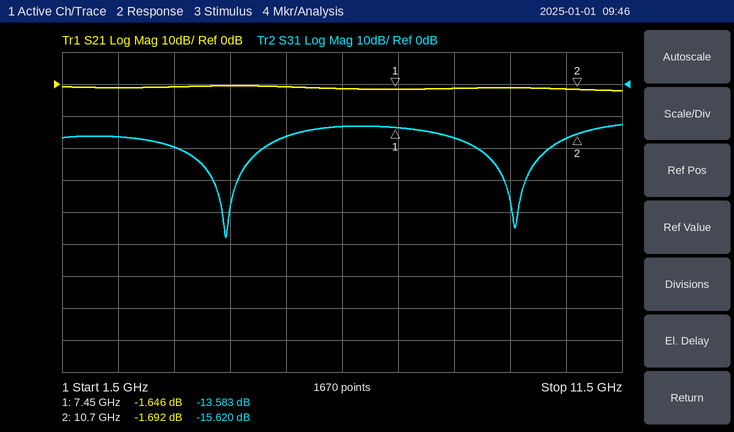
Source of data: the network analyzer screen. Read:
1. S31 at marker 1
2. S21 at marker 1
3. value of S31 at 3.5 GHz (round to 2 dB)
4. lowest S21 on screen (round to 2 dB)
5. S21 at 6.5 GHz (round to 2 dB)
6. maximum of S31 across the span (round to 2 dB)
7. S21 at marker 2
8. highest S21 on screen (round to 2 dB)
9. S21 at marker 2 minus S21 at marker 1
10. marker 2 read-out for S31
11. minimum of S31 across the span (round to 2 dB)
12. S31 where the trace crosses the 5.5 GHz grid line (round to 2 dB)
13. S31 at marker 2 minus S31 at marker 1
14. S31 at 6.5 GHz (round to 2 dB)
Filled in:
-13.583 dB
-1.646 dB
-20 dB
-2 dB
-2 dB
-12 dB
-1.692 dB
0 dB
-0.046 dB
-15.620 dB
-48 dB
-16 dB
-2.037 dB
-14 dB
